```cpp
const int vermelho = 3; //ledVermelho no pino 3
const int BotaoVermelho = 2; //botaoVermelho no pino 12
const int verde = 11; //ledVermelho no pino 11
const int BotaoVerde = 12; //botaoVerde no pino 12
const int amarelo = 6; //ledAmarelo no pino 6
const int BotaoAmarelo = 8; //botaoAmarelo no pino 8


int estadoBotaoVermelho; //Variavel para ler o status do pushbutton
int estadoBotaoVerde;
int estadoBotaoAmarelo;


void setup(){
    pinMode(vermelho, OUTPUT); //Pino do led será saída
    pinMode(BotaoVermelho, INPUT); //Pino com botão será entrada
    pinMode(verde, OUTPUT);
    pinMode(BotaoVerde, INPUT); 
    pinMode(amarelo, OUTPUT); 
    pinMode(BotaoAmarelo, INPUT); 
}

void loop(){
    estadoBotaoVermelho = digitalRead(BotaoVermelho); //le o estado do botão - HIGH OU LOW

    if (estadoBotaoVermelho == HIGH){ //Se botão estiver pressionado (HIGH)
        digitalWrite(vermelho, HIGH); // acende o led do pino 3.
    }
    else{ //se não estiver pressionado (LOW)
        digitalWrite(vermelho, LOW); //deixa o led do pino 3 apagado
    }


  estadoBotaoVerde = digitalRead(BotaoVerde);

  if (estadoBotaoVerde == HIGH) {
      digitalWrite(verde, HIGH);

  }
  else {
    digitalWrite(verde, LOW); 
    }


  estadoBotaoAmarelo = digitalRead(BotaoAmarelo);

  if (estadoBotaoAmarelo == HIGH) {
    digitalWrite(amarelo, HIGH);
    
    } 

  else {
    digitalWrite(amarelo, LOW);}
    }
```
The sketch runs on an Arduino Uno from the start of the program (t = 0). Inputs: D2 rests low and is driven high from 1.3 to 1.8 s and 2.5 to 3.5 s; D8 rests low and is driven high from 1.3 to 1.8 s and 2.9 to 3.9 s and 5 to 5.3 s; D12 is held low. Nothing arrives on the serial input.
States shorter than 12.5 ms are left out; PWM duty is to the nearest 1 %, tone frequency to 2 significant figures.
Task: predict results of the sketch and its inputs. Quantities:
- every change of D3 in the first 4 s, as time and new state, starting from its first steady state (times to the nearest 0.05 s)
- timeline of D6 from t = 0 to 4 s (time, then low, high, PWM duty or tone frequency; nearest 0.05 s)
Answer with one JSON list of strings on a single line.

["0 s low; 1.3 s high; 1.8 s low; 2.5 s high; 3.5 s low", "0 s low; 1.3 s high; 1.8 s low; 2.9 s high; 3.9 s low"]
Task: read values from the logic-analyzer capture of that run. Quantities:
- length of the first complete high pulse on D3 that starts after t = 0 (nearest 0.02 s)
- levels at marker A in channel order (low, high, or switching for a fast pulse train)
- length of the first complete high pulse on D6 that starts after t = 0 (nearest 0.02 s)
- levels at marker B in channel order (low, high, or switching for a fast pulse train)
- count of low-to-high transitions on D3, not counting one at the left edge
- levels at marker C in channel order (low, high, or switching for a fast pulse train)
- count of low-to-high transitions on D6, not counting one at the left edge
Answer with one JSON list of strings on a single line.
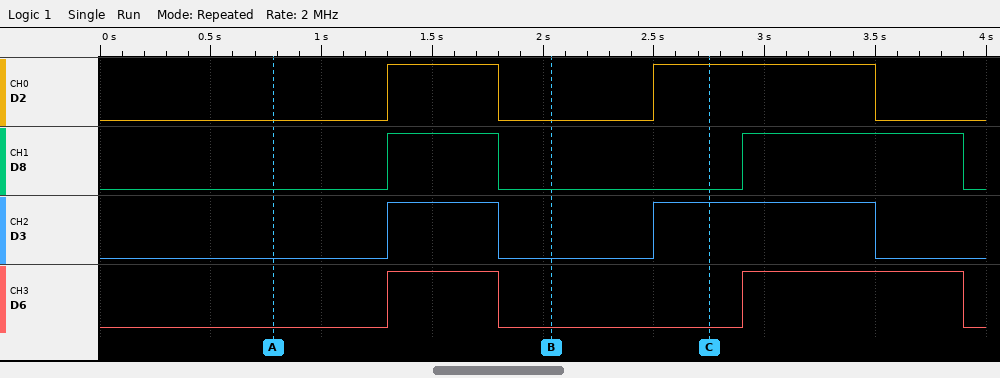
["0.50 s", "D2 low, D8 low, D3 low, D6 low", "0.50 s", "D2 low, D8 low, D3 low, D6 low", "2", "D2 high, D8 low, D3 high, D6 low", "2"]
